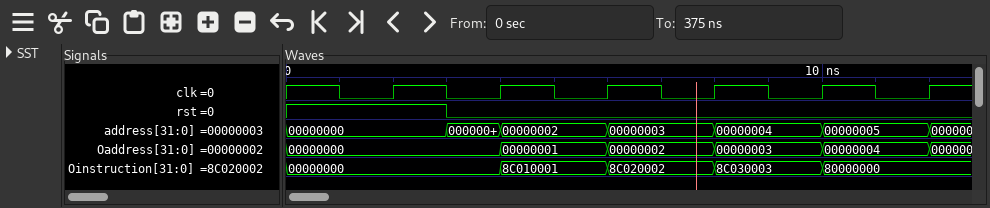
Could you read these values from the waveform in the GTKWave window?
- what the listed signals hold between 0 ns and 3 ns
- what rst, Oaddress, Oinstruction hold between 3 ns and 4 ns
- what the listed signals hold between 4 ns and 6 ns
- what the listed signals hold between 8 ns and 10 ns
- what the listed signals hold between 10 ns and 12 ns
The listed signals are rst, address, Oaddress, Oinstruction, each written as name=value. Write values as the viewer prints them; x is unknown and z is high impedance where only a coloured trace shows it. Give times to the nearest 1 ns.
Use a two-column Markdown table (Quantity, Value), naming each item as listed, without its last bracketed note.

| Quantity | Value |
|---|---|
| what the listed signals hold between 0 ns and 3 ns | rst=1, address=00000000, Oaddress=00000000, Oinstruction=00000000 |
| what rst, Oaddress, Oinstruction hold between 3 ns and 4 ns | rst=0, Oaddress=00000000, Oinstruction=00000000 |
| what the listed signals hold between 4 ns and 6 ns | rst=0, address=00000002, Oaddress=00000001, Oinstruction=8C010001 |
| what the listed signals hold between 8 ns and 10 ns | rst=0, address=00000004, Oaddress=00000003, Oinstruction=8C030003 |
| what the listed signals hold between 10 ns and 12 ns | rst=0, address=00000005, Oaddress=00000004, Oinstruction=80000000 |
